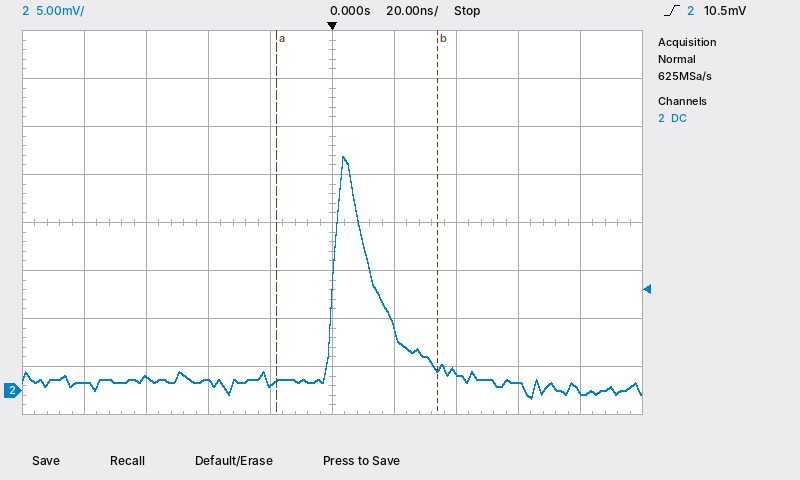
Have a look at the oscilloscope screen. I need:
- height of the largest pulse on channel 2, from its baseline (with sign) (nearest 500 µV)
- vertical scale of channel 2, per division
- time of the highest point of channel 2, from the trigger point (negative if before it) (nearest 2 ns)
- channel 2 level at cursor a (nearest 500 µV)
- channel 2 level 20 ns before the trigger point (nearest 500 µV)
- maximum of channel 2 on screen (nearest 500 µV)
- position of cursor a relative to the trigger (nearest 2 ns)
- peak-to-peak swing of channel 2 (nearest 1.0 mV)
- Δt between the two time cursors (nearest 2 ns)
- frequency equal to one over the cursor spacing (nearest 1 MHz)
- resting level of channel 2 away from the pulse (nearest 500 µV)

+23.5 mV
5 mV
+4 ns
1.0 mV
500 µV
24.5 mV
-18 ns
25.0 mV
52 ns
19 MHz
1.0 mV
